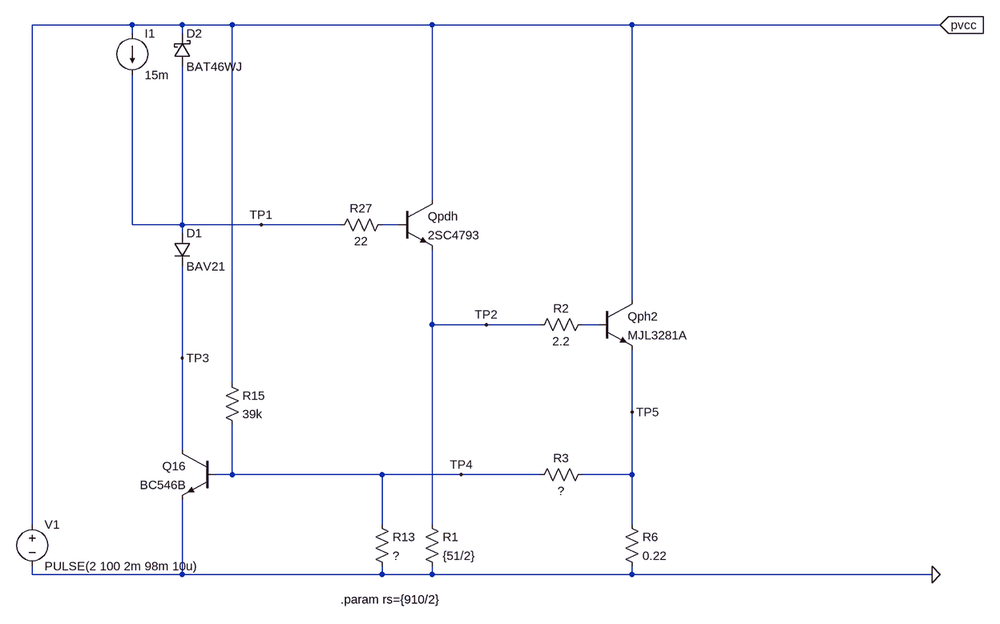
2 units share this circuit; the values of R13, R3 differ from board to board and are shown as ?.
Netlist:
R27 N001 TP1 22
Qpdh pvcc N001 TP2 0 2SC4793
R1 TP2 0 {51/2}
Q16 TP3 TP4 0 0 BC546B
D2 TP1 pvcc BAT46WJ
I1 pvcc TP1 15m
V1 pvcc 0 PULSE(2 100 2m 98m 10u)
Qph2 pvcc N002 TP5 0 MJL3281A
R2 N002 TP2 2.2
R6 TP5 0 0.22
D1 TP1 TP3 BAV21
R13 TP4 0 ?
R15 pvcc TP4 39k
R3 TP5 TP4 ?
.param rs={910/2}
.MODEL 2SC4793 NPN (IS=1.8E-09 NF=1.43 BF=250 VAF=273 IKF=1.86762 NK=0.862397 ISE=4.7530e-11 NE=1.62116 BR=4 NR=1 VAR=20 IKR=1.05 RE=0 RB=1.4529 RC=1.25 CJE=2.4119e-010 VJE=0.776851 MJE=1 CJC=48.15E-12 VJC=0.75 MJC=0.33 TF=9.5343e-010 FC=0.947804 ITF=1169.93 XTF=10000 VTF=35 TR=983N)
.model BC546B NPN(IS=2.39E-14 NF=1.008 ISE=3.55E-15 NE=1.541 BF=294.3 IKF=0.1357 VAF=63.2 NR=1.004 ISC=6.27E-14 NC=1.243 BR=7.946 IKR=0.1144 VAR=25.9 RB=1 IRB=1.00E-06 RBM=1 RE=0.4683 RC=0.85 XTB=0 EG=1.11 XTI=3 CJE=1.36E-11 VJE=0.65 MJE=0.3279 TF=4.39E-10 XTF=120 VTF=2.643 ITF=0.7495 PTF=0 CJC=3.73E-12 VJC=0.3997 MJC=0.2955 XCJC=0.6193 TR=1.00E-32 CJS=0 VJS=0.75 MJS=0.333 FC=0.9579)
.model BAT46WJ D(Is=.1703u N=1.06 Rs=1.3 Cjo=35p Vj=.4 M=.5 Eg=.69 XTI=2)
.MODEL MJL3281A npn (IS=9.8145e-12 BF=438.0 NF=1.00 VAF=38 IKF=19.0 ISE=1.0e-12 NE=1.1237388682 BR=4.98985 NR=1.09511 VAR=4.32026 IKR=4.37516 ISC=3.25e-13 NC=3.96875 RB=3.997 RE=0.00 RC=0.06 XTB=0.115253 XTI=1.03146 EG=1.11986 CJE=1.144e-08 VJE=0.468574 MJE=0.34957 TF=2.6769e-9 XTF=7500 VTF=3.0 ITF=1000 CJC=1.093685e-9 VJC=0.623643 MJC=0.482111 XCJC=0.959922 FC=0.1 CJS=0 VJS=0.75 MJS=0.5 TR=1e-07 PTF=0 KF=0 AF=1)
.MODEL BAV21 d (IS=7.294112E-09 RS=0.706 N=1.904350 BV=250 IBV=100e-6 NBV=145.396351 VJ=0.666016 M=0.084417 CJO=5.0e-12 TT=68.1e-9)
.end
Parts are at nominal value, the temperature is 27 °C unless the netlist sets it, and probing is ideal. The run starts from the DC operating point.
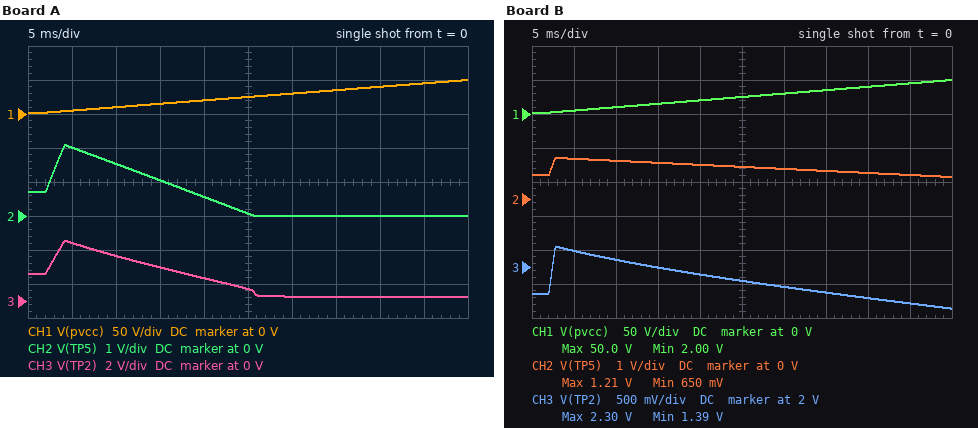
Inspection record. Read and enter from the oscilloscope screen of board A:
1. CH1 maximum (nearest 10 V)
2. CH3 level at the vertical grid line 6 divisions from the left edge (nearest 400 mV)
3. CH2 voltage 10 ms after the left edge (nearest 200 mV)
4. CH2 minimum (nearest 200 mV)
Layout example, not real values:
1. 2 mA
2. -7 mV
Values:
1. 50 V
2. 400 mV
3. 1.6 V
4. 0 V
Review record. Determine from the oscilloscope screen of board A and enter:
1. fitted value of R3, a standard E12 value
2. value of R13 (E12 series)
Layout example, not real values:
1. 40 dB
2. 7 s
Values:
1. 3.9 kΩ
2. 1.8 kΩ
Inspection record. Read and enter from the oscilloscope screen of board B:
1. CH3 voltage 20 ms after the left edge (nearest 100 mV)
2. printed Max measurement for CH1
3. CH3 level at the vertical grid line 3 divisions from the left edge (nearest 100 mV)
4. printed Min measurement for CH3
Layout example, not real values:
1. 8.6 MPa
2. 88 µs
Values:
1. 1.9 V
2. 50.0 V
3. 2.0 V
4. 1.39 V
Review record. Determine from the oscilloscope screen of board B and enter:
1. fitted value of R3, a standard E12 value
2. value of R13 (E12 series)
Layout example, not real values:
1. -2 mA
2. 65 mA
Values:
1. 470 Ω
2. 680 Ω
